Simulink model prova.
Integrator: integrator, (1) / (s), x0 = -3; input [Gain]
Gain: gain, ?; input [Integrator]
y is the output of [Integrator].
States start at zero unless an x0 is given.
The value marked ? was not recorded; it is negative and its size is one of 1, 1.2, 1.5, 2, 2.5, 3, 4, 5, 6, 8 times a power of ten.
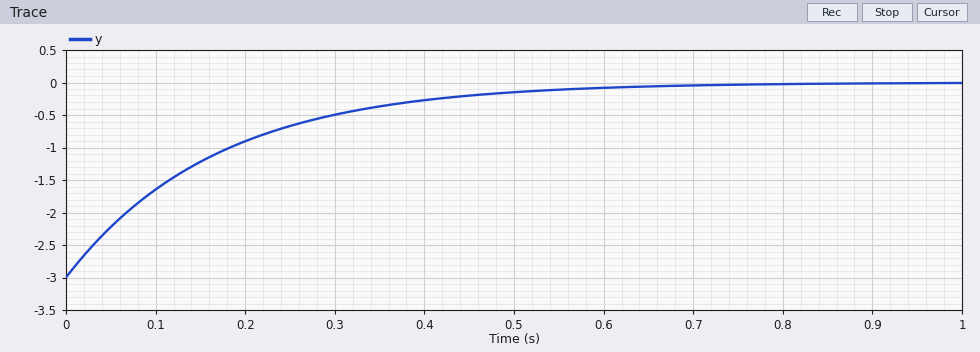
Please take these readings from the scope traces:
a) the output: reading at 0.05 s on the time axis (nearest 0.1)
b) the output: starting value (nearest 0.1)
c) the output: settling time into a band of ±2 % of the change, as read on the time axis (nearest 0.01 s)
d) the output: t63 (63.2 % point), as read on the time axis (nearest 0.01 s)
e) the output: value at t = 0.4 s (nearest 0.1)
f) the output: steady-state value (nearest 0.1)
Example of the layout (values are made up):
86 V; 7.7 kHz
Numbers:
-2.2; -3.0; 0.65 s; 0.17 s; -0.3; 0.0
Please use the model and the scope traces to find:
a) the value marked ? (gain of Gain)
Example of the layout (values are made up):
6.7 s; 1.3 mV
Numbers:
-6
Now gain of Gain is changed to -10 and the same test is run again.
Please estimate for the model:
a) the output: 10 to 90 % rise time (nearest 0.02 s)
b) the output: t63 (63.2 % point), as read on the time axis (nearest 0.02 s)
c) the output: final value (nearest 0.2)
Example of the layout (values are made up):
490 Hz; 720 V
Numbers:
0.22 s; 0.10 s; 0.0
